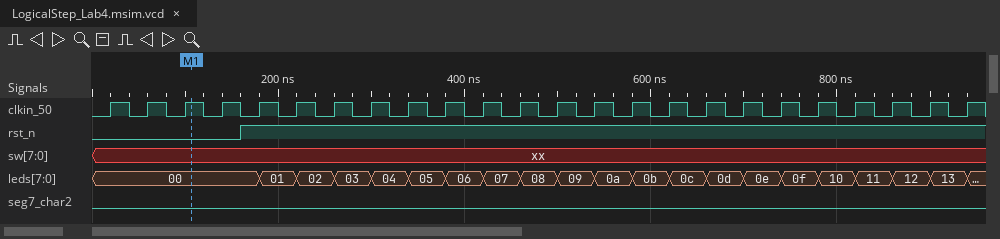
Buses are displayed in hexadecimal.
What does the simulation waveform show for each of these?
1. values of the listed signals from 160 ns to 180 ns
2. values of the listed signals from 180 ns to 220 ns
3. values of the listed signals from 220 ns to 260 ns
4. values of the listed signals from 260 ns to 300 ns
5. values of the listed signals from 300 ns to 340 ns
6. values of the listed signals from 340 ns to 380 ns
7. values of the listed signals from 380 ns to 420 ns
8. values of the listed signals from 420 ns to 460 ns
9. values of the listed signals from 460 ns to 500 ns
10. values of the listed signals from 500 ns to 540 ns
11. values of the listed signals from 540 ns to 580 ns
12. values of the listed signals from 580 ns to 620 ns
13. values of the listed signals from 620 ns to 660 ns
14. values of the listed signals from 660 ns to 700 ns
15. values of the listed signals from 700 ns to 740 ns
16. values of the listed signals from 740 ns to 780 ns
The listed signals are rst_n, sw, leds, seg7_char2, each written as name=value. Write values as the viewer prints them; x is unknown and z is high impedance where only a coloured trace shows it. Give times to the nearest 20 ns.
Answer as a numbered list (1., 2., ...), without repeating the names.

1. rst_n=1, sw=xx, leds=00, seg7_char2=0
2. rst_n=1, sw=xx, leds=01, seg7_char2=0
3. rst_n=1, sw=xx, leds=02, seg7_char2=0
4. rst_n=1, sw=xx, leds=03, seg7_char2=0
5. rst_n=1, sw=xx, leds=04, seg7_char2=0
6. rst_n=1, sw=xx, leds=05, seg7_char2=0
7. rst_n=1, sw=xx, leds=06, seg7_char2=0
8. rst_n=1, sw=xx, leds=07, seg7_char2=0
9. rst_n=1, sw=xx, leds=08, seg7_char2=0
10. rst_n=1, sw=xx, leds=09, seg7_char2=0
11. rst_n=1, sw=xx, leds=0a, seg7_char2=0
12. rst_n=1, sw=xx, leds=0b, seg7_char2=0
13. rst_n=1, sw=xx, leds=0c, seg7_char2=0
14. rst_n=1, sw=xx, leds=0d, seg7_char2=0
15. rst_n=1, sw=xx, leds=0e, seg7_char2=0
16. rst_n=1, sw=xx, leds=0f, seg7_char2=0
